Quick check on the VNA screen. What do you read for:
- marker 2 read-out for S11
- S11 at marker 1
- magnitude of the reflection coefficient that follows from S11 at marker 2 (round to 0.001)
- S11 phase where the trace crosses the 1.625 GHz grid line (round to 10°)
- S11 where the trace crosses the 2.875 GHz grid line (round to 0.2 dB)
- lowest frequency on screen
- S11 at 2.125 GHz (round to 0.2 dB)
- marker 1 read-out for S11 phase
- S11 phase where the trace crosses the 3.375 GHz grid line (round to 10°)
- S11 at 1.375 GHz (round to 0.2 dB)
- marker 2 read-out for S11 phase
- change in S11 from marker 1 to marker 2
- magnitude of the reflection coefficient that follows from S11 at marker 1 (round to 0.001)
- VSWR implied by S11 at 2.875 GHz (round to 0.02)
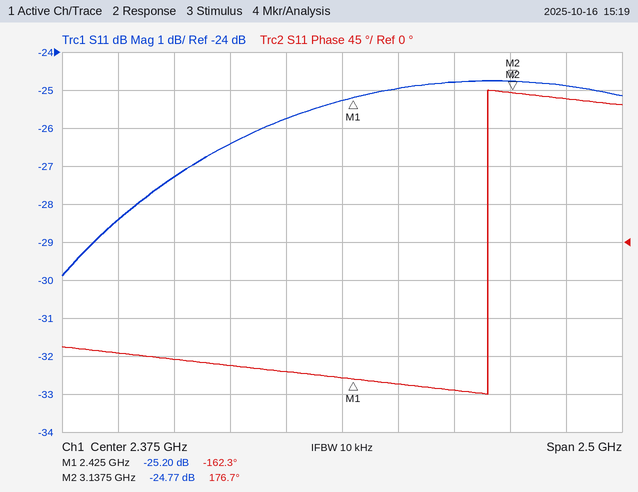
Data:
-24.77 dB
-25.20 dB
0.058
-140°
-24.8 dB
1.125 GHz
-25.8 dB
-162.3°
170°
-28.4 dB
176.7°
0.43 dB
0.055
1.12
